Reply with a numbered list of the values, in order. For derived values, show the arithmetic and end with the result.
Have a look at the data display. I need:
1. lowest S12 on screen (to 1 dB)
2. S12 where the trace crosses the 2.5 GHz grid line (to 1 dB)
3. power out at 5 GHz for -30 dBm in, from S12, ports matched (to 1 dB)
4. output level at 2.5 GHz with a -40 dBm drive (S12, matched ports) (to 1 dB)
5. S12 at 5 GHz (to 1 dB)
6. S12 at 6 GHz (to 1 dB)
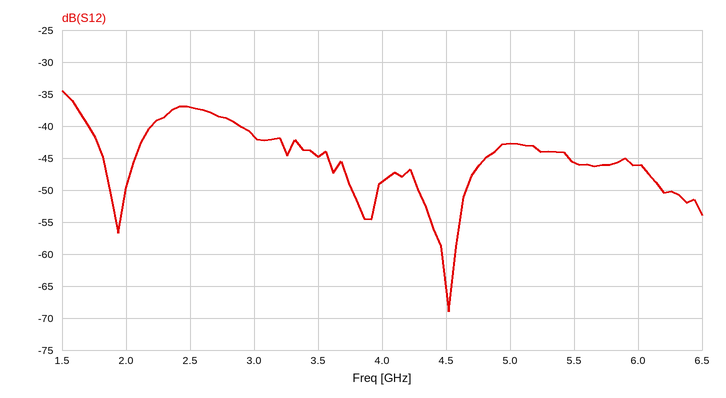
1. -69 dB
2. -37 dB
3. -30 dBm + (-43 dB) = -73 dBm
4. -40 dBm + (-37 dB) = -77 dBm
5. -43 dB
6. -46 dB
